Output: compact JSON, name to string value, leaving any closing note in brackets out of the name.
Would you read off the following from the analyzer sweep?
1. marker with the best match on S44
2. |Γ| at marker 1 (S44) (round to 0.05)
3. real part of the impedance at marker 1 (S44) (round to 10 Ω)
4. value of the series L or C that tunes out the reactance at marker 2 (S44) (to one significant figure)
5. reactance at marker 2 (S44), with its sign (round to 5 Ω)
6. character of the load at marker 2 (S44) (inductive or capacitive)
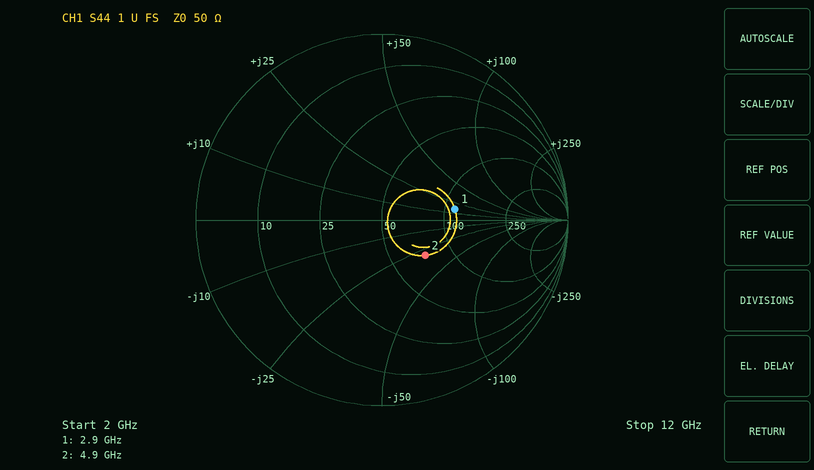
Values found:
{"marker with the best match on S44": "marker 2", "|Γ| at marker 1 (S44)": "0.40", "real part of the impedance at marker 1 (S44)": "110 Ω", "value of the series L or C that tunes out the reactance at marker 2 (S44)": "1.0 nH", "reactance at marker 2 (S44), with its sign": "-30 Ω", "character of the load at marker 2 (S44)": "capacitive"}
